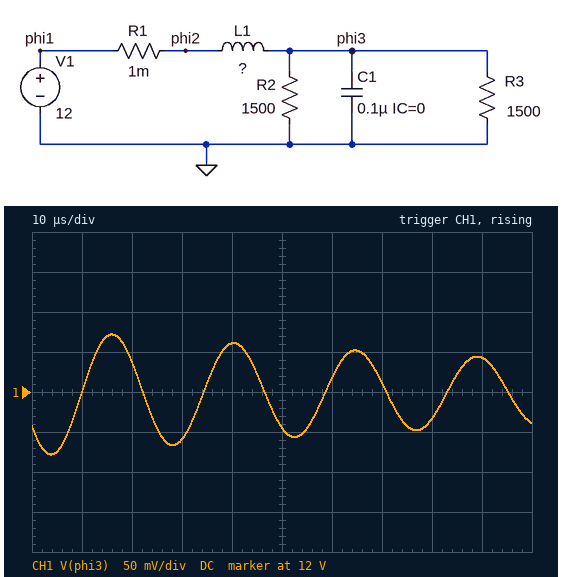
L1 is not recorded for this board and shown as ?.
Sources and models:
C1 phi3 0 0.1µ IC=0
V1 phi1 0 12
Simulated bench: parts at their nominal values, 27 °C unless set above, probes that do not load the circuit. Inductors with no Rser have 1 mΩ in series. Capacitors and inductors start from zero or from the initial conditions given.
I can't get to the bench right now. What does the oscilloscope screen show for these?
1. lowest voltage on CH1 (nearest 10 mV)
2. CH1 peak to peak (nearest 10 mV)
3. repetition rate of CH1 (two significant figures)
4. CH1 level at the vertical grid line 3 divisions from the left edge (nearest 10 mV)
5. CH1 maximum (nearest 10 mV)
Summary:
11.92 V
150 mV
41 kHz
11.94 V
12.07 V
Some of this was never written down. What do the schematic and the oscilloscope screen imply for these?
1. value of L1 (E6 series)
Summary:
150 µH
